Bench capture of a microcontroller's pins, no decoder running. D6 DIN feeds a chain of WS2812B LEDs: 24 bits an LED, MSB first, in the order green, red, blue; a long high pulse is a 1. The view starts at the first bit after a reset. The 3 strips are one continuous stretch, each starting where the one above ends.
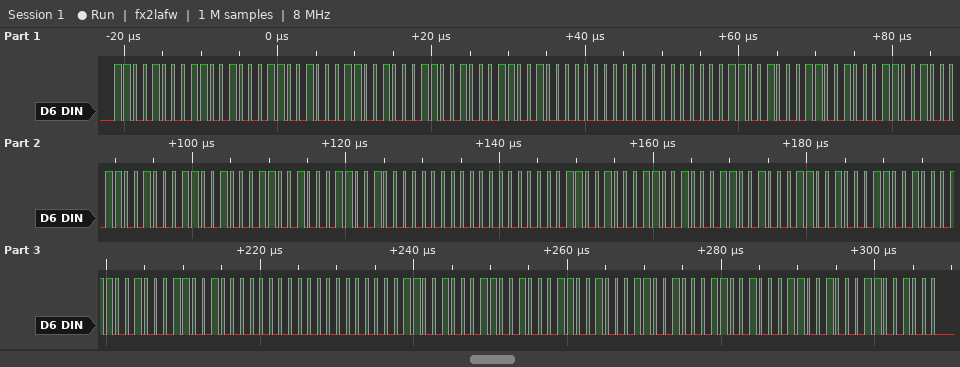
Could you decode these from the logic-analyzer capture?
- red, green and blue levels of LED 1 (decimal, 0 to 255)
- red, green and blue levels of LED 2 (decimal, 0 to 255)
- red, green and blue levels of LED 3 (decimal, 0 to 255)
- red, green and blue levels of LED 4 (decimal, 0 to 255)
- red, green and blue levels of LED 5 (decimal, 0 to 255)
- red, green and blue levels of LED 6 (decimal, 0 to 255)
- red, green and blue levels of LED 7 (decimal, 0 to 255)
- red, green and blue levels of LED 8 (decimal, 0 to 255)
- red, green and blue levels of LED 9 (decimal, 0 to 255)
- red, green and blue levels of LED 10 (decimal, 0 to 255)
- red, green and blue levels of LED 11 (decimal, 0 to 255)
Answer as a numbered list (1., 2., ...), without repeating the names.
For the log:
1. 200, 200, 200
2. 200, 200, 200
3. 0, 0, 200
4. 200, 200, 200
5. 200, 200, 200
6. 0, 0, 200
7. 200, 200, 200
8. 200, 200, 200
9. 0, 0, 200
10. 200, 200, 200
11. 200, 200, 200
